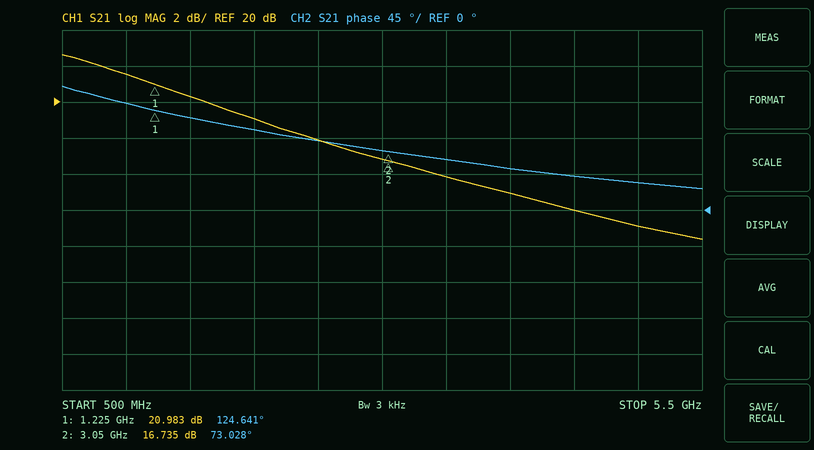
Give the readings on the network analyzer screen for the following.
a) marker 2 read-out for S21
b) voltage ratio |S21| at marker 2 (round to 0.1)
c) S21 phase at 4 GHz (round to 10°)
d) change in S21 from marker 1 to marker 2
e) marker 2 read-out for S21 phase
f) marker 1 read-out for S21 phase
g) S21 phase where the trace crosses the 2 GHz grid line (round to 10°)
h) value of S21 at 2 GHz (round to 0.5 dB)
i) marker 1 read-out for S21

16.735 dB
6.9
50°
-4.248 dB
73.028°
124.641°
100°
19.0 dB
20.983 dB
